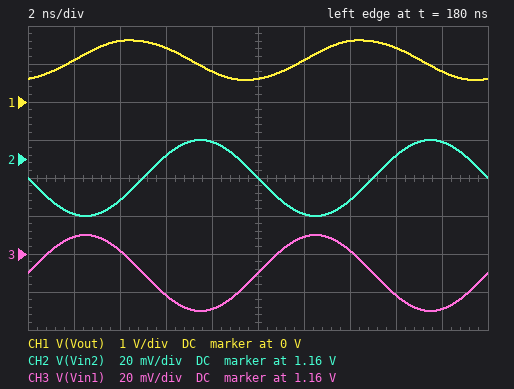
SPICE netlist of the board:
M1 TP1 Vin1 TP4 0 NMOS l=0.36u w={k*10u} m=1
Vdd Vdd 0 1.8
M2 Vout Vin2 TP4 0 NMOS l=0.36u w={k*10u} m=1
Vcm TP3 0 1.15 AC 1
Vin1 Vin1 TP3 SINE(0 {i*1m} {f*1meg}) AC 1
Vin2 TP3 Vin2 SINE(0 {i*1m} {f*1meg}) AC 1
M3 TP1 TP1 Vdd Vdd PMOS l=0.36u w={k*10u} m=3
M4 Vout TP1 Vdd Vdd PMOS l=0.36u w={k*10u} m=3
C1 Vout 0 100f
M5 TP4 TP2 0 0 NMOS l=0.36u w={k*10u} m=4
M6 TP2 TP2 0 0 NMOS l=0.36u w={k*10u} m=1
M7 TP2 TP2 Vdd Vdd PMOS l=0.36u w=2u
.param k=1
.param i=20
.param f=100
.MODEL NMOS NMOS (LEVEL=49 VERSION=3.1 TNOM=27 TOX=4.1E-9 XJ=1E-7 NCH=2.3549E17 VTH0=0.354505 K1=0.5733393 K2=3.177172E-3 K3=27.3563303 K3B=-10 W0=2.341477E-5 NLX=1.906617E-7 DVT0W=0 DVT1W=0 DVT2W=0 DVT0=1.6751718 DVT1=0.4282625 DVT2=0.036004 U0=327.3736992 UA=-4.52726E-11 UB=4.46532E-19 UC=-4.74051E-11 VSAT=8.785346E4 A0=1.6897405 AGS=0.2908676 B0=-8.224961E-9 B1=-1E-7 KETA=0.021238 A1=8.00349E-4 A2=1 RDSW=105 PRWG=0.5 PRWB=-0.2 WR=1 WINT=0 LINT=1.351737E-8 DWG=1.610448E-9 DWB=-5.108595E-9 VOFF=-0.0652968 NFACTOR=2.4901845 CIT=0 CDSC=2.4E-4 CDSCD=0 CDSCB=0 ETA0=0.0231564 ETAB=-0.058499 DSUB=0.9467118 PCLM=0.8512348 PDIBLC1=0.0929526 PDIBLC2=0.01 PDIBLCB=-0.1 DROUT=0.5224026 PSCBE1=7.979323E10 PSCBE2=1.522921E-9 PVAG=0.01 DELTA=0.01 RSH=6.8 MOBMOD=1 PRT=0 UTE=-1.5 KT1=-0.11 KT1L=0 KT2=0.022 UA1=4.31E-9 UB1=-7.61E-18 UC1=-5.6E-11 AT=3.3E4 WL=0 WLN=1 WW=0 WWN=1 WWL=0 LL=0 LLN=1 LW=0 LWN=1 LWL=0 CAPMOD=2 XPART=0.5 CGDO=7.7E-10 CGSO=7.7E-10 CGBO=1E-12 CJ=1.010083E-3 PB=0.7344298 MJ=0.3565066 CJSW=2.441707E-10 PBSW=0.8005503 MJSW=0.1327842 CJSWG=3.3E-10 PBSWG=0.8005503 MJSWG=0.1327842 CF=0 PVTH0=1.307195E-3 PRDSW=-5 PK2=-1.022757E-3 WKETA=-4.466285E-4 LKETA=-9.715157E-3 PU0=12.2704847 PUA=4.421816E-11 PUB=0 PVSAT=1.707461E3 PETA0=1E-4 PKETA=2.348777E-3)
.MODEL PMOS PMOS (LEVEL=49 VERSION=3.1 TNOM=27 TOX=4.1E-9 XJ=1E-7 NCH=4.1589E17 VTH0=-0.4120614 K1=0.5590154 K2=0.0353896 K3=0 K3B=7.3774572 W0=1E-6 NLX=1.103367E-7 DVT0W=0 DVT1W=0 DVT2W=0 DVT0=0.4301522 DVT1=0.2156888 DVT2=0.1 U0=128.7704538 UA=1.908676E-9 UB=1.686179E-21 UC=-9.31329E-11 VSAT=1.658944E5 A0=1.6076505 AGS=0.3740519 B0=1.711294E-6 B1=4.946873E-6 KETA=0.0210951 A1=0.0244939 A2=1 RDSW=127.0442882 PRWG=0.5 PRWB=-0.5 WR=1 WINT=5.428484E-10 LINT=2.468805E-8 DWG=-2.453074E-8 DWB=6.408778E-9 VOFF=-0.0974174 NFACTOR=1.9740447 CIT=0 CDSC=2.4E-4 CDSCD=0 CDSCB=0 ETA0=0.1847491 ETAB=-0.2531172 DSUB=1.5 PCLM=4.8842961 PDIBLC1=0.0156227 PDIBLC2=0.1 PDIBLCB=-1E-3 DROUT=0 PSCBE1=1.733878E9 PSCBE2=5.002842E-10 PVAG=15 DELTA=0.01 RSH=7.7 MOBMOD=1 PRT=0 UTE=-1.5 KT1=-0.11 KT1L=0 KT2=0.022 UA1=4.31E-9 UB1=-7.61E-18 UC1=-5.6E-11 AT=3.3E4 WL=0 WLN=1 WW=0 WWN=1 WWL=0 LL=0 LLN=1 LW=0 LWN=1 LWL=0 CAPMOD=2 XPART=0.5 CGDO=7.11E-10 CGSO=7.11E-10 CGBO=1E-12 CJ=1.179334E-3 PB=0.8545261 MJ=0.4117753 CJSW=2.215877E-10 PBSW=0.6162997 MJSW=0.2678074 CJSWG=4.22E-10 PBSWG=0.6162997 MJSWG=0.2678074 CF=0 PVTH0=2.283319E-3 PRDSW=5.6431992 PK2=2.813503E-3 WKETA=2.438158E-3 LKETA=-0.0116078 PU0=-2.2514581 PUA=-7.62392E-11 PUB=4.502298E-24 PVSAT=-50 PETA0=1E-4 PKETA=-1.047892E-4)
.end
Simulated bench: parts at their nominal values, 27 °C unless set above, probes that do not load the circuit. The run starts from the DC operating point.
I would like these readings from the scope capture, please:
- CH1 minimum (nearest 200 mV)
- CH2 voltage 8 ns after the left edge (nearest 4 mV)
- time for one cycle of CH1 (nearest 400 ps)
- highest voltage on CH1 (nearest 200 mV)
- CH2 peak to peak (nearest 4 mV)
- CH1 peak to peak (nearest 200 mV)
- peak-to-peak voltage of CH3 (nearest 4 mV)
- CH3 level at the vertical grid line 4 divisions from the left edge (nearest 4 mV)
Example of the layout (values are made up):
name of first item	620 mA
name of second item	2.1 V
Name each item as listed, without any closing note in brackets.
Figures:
CH1 minimum	600 mV
CH2 voltage 8 ns after the left edge	1.168 V
time for one cycle of CH1	10.0 ns
highest voltage on CH1	1.6 V
CH2 peak to peak	40 mV
CH1 peak to peak	1.0 V
peak-to-peak voltage of CH3	40 mV
CH3 level at the vertical grid line 4 divisions from the left edge	1.132 V
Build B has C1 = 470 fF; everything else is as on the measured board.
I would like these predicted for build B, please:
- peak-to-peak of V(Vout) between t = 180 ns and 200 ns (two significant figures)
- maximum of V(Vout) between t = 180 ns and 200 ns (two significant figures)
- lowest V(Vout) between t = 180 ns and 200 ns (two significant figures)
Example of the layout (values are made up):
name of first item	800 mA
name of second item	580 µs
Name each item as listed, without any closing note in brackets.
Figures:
peak-to-peak of V(Vout) between t = 180 ns and 200 ns	340 mV
maximum of V(Vout) between t = 180 ns and 200 ns	1.3 V
lowest V(Vout) between t = 180 ns and 200 ns	940 mV
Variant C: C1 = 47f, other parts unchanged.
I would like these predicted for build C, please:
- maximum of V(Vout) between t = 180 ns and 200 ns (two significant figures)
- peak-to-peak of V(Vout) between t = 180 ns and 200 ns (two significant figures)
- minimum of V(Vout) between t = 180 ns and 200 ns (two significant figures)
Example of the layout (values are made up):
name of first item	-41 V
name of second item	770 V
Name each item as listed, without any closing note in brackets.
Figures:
maximum of V(Vout) between t = 180 ns and 200 ns	1.7 V
peak-to-peak of V(Vout) between t = 180 ns and 200 ns	1.2 V
minimum of V(Vout) between t = 180 ns and 200 ns	500 mV
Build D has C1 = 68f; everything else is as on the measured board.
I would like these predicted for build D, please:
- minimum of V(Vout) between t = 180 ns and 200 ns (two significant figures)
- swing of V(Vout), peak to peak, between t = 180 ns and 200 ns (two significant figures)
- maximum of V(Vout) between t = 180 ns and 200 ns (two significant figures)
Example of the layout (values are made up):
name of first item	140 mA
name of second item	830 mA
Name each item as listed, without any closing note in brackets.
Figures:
minimum of V(Vout) between t = 180 ns and 200 ns	520 mV
swing of V(Vout), peak to peak, between t = 180 ns and 200 ns	1.1 V
maximum of V(Vout) between t = 180 ns and 200 ns	1.7 V
